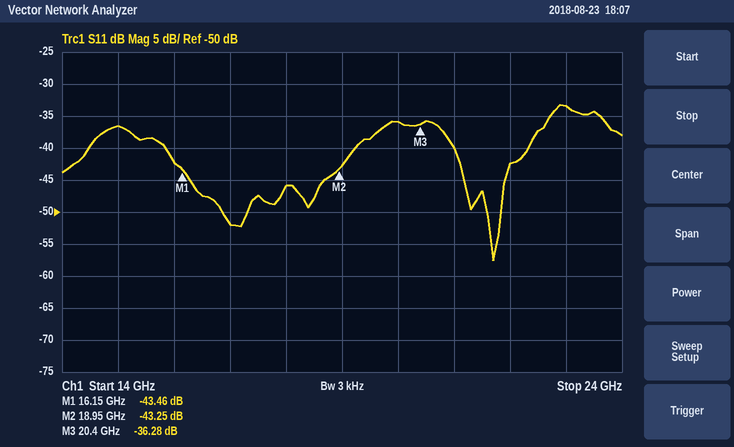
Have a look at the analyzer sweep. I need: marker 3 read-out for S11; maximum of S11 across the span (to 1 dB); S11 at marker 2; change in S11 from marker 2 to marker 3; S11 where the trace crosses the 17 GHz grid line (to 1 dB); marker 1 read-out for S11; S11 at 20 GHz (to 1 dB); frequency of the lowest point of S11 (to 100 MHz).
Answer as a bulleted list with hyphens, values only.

- -36.28 dB
- -33 dB
- -43.25 dB
- 6.97 dB
- -52 dB
- -43.46 dB
- -36 dB
- 21.7 GHz
